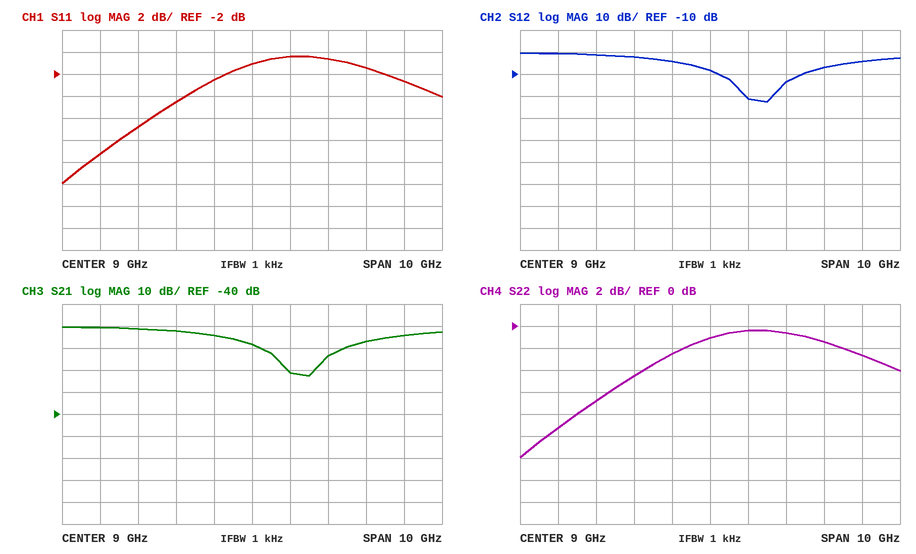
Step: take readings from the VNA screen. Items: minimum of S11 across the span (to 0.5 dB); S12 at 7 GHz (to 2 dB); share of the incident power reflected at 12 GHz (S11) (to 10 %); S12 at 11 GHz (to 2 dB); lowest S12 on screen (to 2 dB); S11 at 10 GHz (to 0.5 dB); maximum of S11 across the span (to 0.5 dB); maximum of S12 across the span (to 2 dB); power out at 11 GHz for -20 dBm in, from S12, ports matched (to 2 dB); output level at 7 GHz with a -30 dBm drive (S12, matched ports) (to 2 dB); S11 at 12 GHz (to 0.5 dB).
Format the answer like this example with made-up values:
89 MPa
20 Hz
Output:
-12.0 dB
-2 dB
70 %
-14 dB
-22 dB
-0.5 dB
-0.5 dB
0 dB
-34 dBm
-32 dBm
-1.5 dB
